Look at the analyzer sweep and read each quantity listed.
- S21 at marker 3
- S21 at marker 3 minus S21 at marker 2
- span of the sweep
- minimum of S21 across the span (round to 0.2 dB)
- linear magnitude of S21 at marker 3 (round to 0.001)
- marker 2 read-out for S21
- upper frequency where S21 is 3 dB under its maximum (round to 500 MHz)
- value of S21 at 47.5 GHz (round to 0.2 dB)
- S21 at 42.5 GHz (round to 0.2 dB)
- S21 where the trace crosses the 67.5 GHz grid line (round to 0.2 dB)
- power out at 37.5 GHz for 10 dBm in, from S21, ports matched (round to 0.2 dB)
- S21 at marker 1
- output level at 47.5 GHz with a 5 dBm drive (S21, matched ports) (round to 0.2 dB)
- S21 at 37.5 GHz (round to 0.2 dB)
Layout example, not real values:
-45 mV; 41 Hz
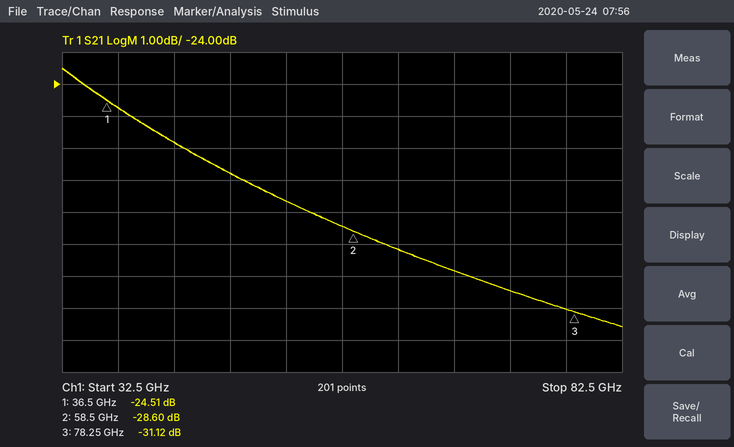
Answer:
-31.12 dB; -2.52 dB; 50 GHz; -31.6 dB; 0.028; -28.60 dB; 46.0 GHz; -26.8 dB; -25.8 dB; -29.8 dB; -14.8 dBm; -24.51 dB; -21.8 dBm; -24.8 dB
